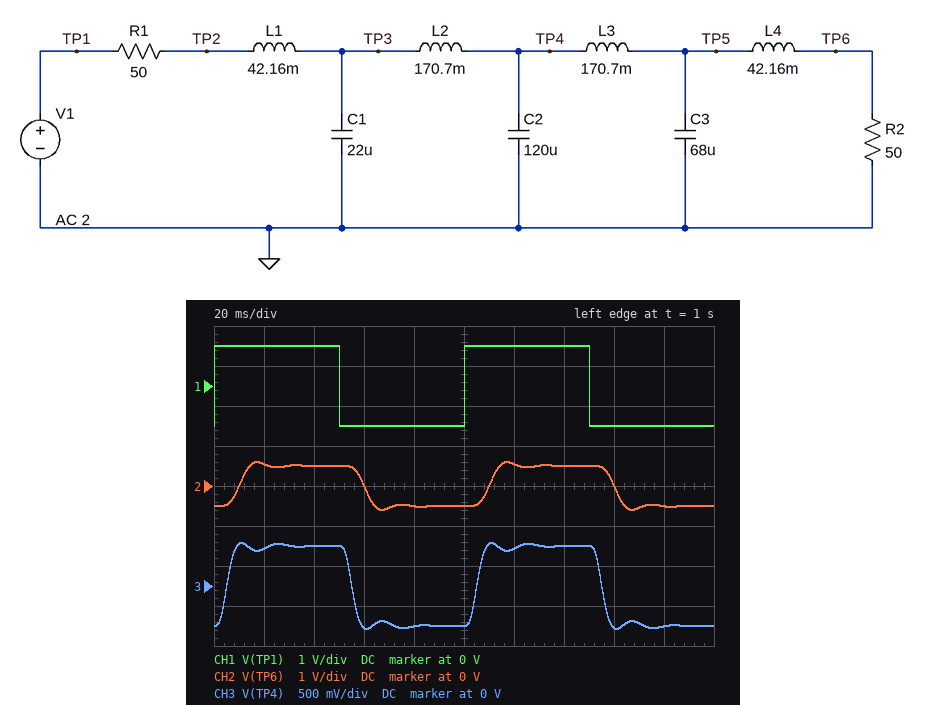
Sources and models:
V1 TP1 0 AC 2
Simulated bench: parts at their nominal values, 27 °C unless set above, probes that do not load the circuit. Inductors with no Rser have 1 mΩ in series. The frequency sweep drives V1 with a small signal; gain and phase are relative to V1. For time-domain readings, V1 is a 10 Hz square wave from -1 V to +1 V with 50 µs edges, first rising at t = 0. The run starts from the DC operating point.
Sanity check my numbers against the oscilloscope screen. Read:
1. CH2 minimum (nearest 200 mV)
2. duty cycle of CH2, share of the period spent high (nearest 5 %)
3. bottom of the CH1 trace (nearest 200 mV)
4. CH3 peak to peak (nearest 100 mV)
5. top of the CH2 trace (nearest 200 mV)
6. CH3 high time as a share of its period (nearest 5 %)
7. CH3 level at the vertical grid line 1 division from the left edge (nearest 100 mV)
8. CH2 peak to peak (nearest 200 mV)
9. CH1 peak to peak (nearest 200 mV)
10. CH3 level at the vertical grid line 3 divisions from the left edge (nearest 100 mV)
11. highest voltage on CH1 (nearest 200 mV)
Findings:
-600 mV
50 %
-1.0 V
1.1 V
600 mV
50 %
500 mV
1.2 V
2.0 V
-500 mV
1.0 V
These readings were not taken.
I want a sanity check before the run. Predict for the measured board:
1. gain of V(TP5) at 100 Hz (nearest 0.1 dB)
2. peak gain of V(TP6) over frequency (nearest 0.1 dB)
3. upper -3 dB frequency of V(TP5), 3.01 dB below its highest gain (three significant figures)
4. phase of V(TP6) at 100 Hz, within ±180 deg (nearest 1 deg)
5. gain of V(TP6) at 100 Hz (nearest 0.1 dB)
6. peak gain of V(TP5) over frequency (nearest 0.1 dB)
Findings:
-24.8 dB
-6.0 dB
63.8 Hz
-3 deg
-25.8 dB
-6.0 dB
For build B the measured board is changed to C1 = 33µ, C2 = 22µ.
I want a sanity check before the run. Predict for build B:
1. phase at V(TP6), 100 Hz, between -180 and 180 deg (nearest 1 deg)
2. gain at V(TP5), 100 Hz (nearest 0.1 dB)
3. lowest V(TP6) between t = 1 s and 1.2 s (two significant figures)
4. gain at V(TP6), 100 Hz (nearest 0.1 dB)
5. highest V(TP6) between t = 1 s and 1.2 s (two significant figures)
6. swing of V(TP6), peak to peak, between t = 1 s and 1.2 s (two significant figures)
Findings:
105 deg
-10.5 dB
-560 mV
-11.5 dB
560 mV
1.1 V
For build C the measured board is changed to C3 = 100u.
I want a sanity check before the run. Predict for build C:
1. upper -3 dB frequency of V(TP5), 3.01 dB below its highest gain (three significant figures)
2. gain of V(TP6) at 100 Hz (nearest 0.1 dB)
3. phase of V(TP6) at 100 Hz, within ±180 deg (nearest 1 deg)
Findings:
61.8 Hz
-30.1 dB
-17 deg
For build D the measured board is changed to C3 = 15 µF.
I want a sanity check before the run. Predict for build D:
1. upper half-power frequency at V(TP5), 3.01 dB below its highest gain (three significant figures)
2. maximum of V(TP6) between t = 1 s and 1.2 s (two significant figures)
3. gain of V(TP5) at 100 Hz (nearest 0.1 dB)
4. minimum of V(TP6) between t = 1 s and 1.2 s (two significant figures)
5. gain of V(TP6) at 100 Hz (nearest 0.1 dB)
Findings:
51.5 Hz
580 mV
-21.0 dB
-580 mV
-22.1 dB
